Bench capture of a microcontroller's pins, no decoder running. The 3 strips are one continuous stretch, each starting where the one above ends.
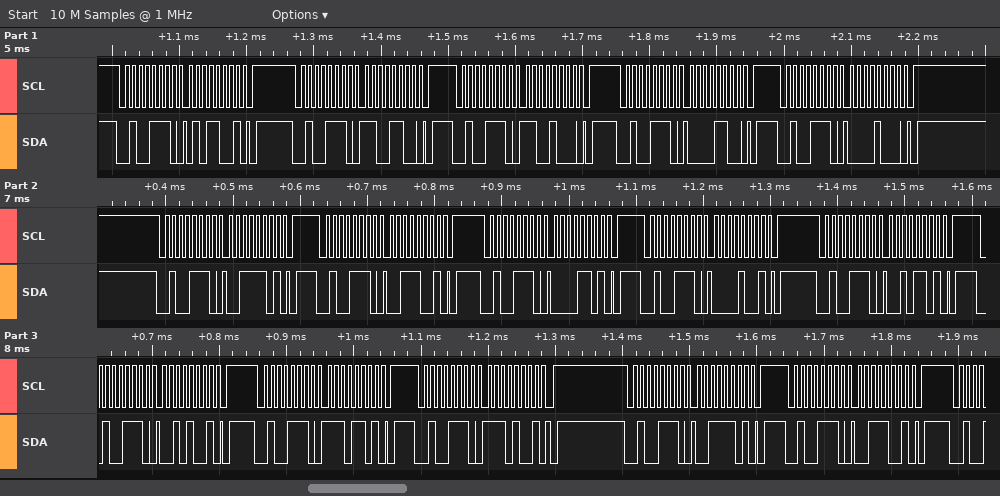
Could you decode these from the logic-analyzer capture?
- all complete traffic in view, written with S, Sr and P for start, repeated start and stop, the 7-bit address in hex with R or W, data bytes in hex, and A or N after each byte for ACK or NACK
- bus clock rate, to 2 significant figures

S 27W A 59 A P S 27W A CC A P S 27W A C8 A P S 27W A 0C A P S 27W A 08 A P S 27W A 3D A P S 27W A 39 A P S 27W A 0D A P S 27W A 09 A P S 27W A 2D A P S 27W A 29 A P S 27W A ED A P S 27W A E9 A P S 27W A 3D A P S 27W A 39 A P
100 kHz
